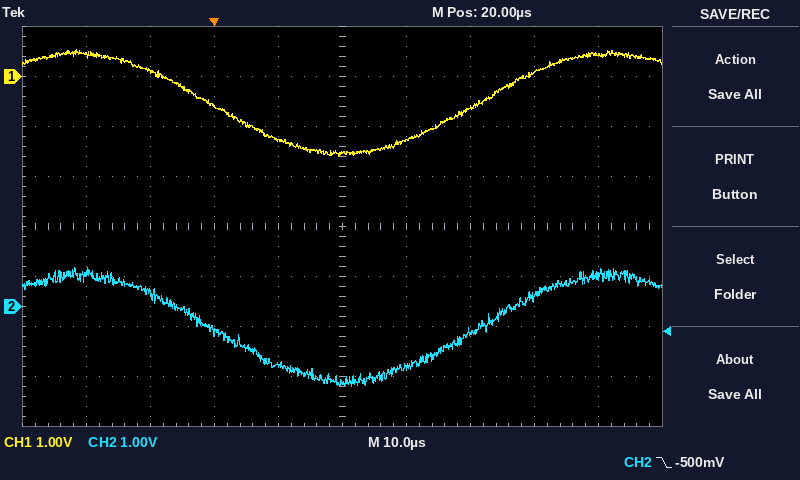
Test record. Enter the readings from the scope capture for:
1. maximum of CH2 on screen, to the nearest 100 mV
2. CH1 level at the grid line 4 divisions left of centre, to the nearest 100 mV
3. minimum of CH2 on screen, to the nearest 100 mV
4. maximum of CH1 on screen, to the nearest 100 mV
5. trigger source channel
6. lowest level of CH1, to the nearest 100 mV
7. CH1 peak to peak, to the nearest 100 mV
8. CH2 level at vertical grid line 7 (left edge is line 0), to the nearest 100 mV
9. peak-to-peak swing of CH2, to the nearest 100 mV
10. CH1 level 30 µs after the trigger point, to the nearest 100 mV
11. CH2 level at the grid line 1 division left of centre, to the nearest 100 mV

800 mV
400 mV
-1.6 V
500 mV
CH2
-1.6 V
2.1 V
-500 mV
2.4 V
-1.3 V
-1.2 V
